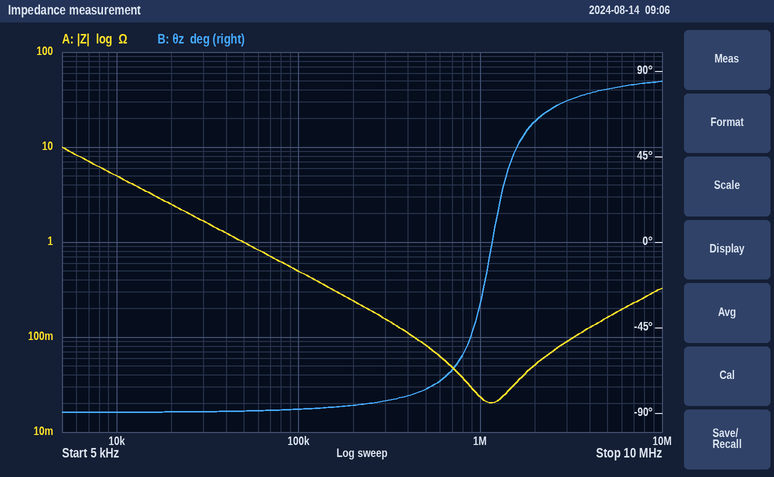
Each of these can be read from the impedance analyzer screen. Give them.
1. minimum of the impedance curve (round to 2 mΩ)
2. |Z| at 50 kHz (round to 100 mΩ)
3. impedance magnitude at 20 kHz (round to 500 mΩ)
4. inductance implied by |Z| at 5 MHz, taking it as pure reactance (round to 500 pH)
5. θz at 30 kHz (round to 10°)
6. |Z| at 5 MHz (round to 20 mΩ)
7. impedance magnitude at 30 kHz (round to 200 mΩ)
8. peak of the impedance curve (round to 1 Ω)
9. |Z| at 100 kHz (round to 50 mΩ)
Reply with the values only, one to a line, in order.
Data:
20 mΩ
1.0 Ω
2.5 Ω
5.0 nH
-90°
160 mΩ
1.6 Ω
10 Ω
500 mΩ
